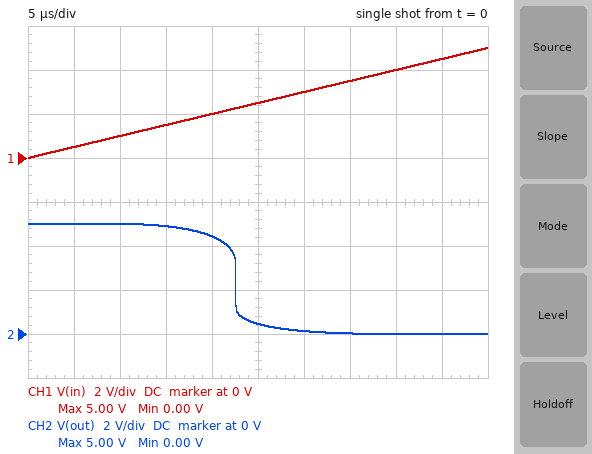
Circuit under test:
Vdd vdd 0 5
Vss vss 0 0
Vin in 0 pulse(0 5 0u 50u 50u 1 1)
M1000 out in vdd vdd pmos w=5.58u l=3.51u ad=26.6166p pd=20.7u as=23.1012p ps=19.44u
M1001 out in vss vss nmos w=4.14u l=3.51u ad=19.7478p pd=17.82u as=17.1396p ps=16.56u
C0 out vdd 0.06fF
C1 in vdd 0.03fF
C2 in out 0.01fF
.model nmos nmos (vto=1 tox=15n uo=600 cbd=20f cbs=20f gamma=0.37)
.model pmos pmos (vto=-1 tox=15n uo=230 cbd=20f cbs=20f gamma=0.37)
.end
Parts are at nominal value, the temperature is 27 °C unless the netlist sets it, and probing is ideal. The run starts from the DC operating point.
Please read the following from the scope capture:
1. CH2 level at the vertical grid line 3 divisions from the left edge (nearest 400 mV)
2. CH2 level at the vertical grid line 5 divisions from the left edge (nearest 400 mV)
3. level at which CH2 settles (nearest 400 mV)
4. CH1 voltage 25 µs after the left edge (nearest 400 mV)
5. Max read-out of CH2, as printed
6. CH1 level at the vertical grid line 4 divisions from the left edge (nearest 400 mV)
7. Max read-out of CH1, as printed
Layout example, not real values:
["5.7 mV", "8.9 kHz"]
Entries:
["4.8 V", "400 mV", "0 V", "2.4 V", "5.00 V", "2.0 V", "5.00 V"]
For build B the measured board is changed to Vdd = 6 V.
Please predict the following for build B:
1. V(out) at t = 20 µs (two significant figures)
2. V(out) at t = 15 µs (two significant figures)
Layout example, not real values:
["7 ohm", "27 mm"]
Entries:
["5.7 V", "5.9 V"]
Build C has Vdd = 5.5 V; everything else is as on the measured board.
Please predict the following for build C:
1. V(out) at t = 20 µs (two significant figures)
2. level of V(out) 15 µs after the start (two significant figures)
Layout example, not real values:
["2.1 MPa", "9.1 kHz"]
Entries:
["5.1 V", "5.4 V"]
